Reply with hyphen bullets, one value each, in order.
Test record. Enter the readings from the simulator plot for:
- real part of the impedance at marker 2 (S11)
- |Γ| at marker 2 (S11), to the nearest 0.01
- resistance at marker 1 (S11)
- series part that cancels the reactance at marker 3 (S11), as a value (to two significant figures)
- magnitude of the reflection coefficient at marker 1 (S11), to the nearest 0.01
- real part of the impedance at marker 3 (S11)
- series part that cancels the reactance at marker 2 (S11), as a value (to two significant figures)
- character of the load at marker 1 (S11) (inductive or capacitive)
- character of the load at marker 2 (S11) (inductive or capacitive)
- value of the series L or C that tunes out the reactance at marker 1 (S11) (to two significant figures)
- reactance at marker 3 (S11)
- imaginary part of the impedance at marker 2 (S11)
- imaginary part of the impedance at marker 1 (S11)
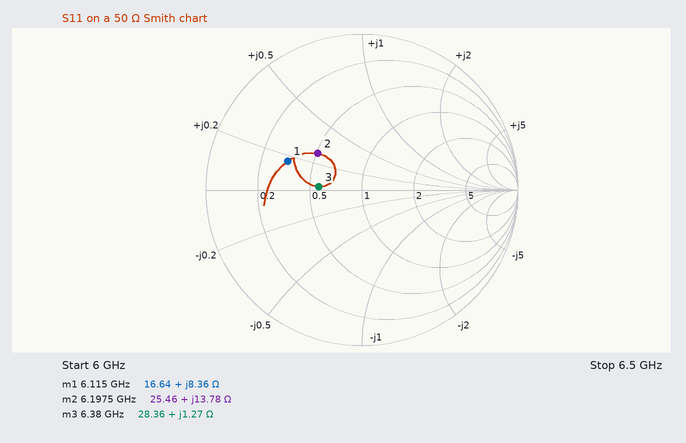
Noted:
- 25.46 Ω
- 0.37
- 16.64 Ω
- 20 pF
- 0.51
- 28.36 Ω
- 1.9 pF
- inductive
- inductive
- 3.1 pF
- +1.27 Ω
- +13.78 Ω
- +8.36 Ω
